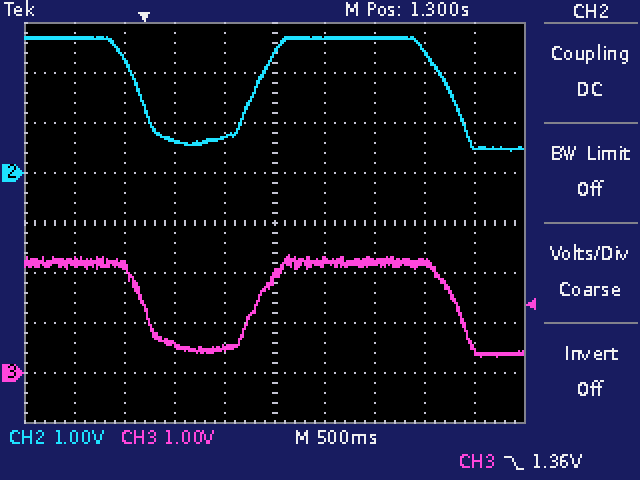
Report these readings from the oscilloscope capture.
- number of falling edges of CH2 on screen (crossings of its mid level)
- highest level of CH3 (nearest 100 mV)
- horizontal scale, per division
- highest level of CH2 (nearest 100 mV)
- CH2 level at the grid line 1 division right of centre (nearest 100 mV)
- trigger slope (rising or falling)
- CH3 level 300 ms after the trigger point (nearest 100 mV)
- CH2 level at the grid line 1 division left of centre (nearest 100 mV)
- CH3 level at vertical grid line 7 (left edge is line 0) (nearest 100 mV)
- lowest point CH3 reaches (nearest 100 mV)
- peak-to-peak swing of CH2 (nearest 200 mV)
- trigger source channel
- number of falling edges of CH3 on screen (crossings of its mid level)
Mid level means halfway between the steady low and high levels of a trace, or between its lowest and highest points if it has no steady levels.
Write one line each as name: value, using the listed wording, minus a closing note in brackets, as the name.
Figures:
number of falling edges of CH2 on screen: 2
highest level of CH3: 2.4 V
horizontal scale, per division: 500 ms
highest level of CH2: 2.7 V
CH2 level at the grid line 1 division right of centre: 2.7 V
trigger slope: falling
CH3 level 300 ms after the trigger point: 600 mV
CH2 level at the grid line 1 division left of centre: 700 mV
CH3 level at vertical grid line 7 (left edge is line 0): 2.2 V
lowest point CH3 reaches: 300 mV
peak-to-peak swing of CH2: 2.2 V
trigger source channel: CH3
number of falling edges of CH3 on screen: 2
